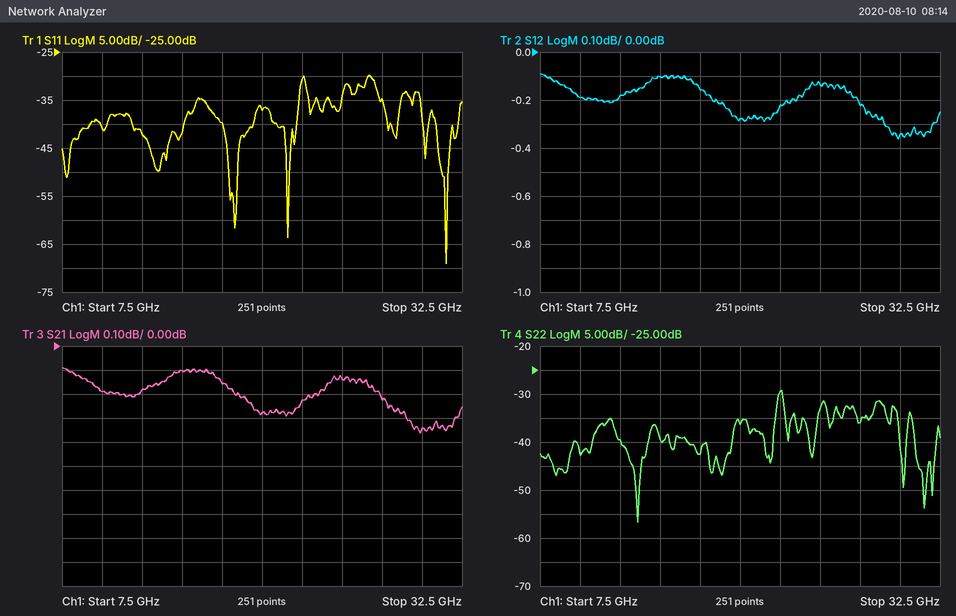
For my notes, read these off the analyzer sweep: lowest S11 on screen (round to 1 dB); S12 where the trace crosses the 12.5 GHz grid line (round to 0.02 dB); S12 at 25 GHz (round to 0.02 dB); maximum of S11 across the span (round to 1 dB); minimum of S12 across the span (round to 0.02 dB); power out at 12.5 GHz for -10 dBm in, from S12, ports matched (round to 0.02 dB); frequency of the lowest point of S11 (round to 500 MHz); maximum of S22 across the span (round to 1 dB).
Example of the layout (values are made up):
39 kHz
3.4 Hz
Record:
-69 dB
-0.18 dB
-0.14 dB
-30 dB
-0.36 dB
-10.18 dBm
31.5 GHz
-29 dB
